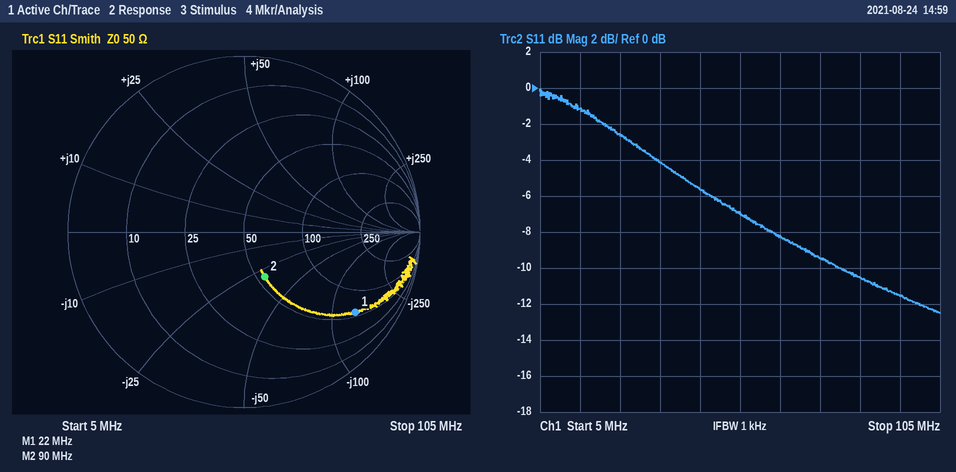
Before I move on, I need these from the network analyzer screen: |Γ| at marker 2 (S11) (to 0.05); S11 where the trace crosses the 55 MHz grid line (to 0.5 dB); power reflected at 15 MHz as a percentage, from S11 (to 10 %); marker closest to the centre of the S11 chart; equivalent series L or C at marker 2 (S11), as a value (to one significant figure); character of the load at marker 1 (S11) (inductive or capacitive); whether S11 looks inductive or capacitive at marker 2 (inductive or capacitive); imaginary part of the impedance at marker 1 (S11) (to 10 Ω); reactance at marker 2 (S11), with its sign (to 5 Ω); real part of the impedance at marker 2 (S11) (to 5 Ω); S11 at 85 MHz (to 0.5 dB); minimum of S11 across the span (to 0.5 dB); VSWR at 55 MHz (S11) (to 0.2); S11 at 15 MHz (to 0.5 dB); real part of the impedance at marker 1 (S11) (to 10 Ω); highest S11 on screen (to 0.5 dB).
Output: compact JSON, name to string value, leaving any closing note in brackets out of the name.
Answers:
{"|Γ| at marker 2 (S11)": "0.30", "S11 where the trace crosses the 55 MHz grid line": "-7.0 dB", "power reflected at 15 MHz as a percentage, from S11": "80 %", "marker closest to the centre of the S11 chart": "marker 2", "equivalent series L or C at marker 2 (S11), as a value": "60 pF", "character of the load at marker 1 (S11)": "capacitive", "whether S11 looks inductive or capacitive at marker 2": "capacitive", "imaginary part of the impedance at marker 1 (S11)": "-130 Ω", "reactance at marker 2 (S11), with its sign": "-30 Ω", "real part of the impedance at marker 2 (S11)": "55 Ω", "S11 at 85 MHz": "-10.5 dB", "minimum of S11 across the span": "-12.5 dB", "VSWR at 55 MHz (S11)": "2.6", "S11 at 15 MHz": "-1.0 dB", "real part of the impedance at marker 1 (S11)": "60 Ω", "highest S11 on screen": "0.0 dB"}
